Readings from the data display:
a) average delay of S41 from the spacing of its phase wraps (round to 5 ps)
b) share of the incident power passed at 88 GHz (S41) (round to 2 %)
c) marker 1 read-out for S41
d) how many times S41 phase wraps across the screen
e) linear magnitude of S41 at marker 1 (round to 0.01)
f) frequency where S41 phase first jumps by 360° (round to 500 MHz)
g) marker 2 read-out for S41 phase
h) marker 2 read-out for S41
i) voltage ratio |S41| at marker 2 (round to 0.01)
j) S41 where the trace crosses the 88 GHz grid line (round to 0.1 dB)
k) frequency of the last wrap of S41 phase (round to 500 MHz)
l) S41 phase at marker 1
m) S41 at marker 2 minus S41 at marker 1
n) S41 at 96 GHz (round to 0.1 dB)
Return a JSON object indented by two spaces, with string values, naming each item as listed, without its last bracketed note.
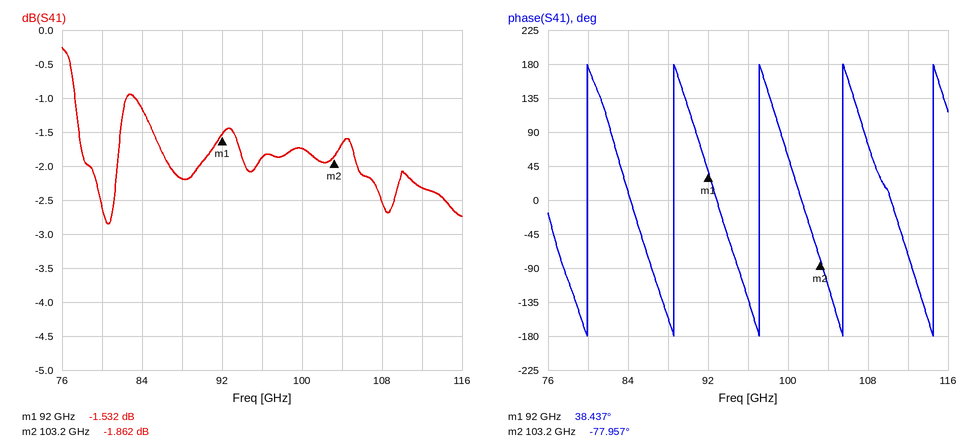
{
  "average delay of S41 from the spacing of its phase wraps": "115 ps",
  "share of the incident power passed at 88 GHz (S41)": "60 %",
  "marker 1 read-out for S41": "-1.532 dB",
  "how many times S41 phase wraps across the screen": "5",
  "linear magnitude of S41 at marker 1": "0.84",
  "frequency where S41 phase first jumps by 360°": "80.0 GHz",
  "marker 2 read-out for S41 phase": "-77.957°",
  "marker 2 read-out for S41": "-1.862 dB",
  "voltage ratio |S41| at marker 2": "0.81",
  "S41 where the trace crosses the 88 GHz grid line": "-2.2 dB",
  "frequency of the last wrap of S41 phase": "114.5 GHz",
  "S41 phase at marker 1": "38.437°",
  "S41 at marker 2 minus S41 at marker 1": "-0.330 dB",
  "S41 at 96 GHz": "-1.9 dB"
}
